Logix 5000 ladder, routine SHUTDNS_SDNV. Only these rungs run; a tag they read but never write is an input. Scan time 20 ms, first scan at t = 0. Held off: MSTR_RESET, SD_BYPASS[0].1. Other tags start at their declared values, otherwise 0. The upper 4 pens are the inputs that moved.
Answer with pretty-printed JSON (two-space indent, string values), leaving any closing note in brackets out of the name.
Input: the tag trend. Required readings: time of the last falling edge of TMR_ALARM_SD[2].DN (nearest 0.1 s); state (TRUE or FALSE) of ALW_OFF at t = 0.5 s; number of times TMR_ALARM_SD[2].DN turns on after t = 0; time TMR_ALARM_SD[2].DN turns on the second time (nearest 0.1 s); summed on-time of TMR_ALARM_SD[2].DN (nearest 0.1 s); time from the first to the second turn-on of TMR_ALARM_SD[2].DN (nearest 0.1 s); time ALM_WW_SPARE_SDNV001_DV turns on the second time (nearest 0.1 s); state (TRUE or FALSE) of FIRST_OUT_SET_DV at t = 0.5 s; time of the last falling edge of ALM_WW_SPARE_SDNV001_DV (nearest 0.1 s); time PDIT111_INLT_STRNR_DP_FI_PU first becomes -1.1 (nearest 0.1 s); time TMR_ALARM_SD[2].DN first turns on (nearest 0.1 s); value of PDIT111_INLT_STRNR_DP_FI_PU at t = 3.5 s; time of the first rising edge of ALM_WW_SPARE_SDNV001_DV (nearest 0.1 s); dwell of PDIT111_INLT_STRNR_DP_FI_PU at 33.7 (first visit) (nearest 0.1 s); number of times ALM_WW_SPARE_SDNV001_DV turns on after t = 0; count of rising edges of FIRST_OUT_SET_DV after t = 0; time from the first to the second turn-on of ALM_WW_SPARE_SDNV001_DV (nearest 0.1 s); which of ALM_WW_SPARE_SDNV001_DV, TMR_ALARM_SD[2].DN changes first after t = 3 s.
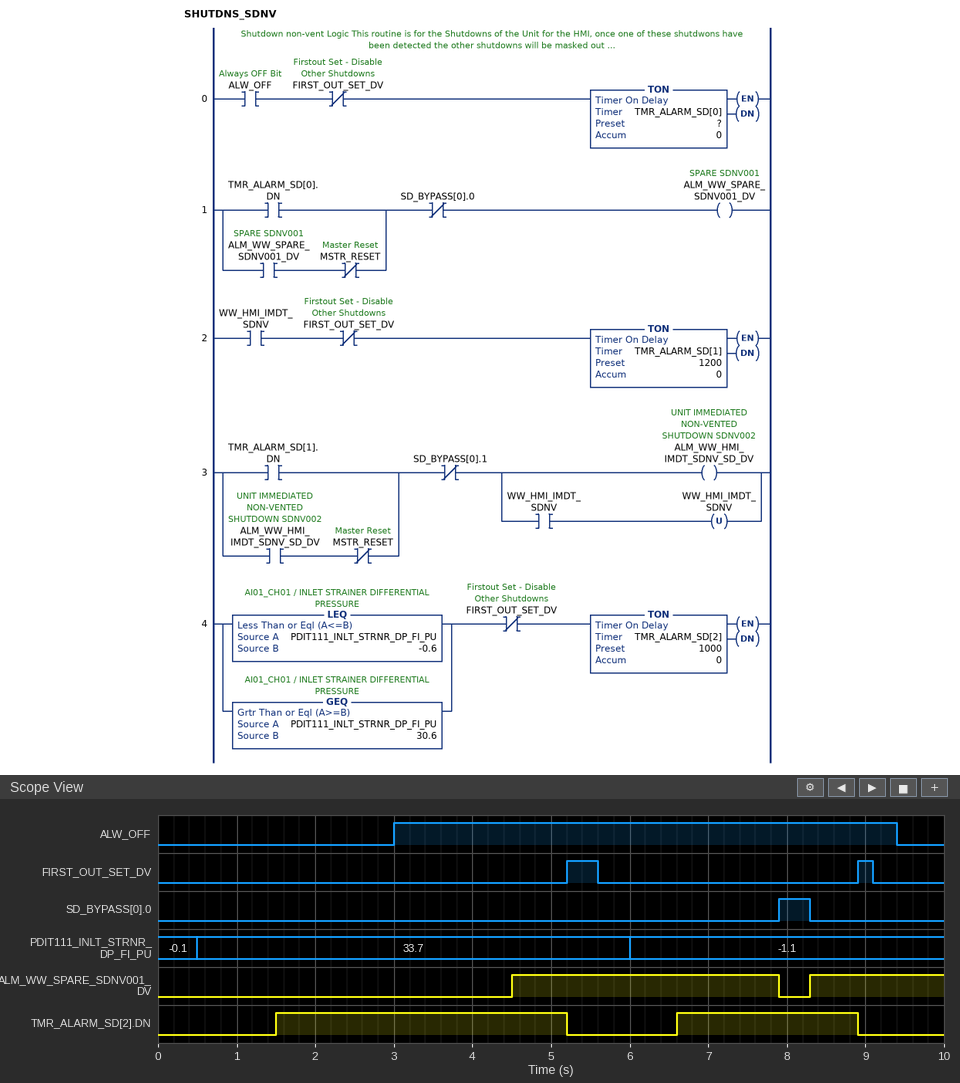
{
  "time of the last falling edge of TMR_ALARM_SD[2].DN": "8.9 s",
  "state (TRUE or FALSE) of ALW_OFF at t = 0.5 s": "FALSE",
  "number of times TMR_ALARM_SD[2].DN turns on after t = 0": "2",
  "time TMR_ALARM_SD[2].DN turns on the second time": "6.6 s",
  "summed on-time of TMR_ALARM_SD[2].DN": "6.0 s",
  "time from the first to the second turn-on of TMR_ALARM_SD[2].DN": "5.1 s",
  "time ALM_WW_SPARE_SDNV001_DV turns on the second time": "8.3 s",
  "state (TRUE or FALSE) of FIRST_OUT_SET_DV at t = 0.5 s": "FALSE",
  "time of the last falling edge of ALM_WW_SPARE_SDNV001_DV": "7.9 s",
  "time PDIT111_INLT_STRNR_DP_FI_PU first becomes -1.1": "6.0 s",
  "time TMR_ALARM_SD[2].DN first turns on": "1.5 s",
  "value of PDIT111_INLT_STRNR_DP_FI_PU at t = 3.5 s": "33.7",
  "time of the first rising edge of ALM_WW_SPARE_SDNV001_DV": "4.5 s",
  "dwell of PDIT111_INLT_STRNR_DP_FI_PU at 33.7 (first visit)": "5.5 s",
  "number of times ALM_WW_SPARE_SDNV001_DV turns on after t = 0": "2",
  "count of rising edges of FIRST_OUT_SET_DV after t = 0": "2",
  "time from the first to the second turn-on of ALM_WW_SPARE_SDNV001_DV": "3.8 s",
  "which of ALM_WW_SPARE_SDNV001_DV, TMR_ALARM_SD[2].DN changes first after t = 3 s": "ALM_WW_SPARE_SDNV001_DV"
}
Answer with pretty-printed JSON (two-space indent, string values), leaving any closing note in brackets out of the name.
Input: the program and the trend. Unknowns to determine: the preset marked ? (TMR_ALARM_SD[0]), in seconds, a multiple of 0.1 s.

{
  "the preset marked ? (TMR_ALARM_SD[0]), in seconds, a multiple of 0.1 s": "1.5 s"
}
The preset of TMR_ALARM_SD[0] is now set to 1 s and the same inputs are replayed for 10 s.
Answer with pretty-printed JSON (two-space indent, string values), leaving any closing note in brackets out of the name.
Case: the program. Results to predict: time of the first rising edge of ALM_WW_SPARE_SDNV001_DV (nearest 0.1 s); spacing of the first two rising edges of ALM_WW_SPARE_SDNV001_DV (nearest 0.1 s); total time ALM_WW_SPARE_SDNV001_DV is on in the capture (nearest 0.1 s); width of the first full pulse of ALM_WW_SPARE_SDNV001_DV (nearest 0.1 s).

{
  "time of the first rising edge of ALM_WW_SPARE_SDNV001_DV": "4.0 s",
  "spacing of the first two rising edges of ALM_WW_SPARE_SDNV001_DV": "4.3 s",
  "total time ALM_WW_SPARE_SDNV001_DV is on in the capture": "5.6 s",
  "width of the first full pulse of ALM_WW_SPARE_SDNV001_DV": "3.9 s"
}
